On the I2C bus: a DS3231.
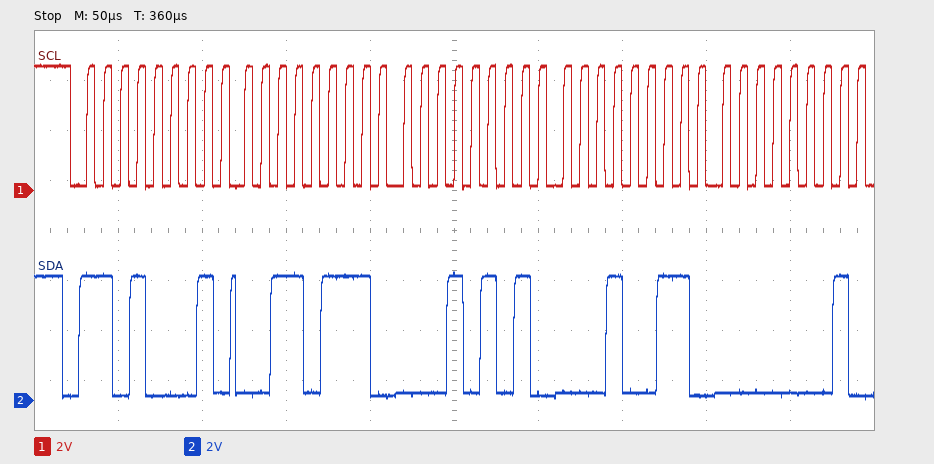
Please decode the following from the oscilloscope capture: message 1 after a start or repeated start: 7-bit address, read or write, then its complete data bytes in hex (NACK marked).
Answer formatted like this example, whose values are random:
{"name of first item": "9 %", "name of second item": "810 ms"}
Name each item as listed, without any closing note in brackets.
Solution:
{"message 1 after a start or repeated start: 7-bit address, read or write, then its complete data bytes in hex": "0x68 read: 37 15 13 01"}
